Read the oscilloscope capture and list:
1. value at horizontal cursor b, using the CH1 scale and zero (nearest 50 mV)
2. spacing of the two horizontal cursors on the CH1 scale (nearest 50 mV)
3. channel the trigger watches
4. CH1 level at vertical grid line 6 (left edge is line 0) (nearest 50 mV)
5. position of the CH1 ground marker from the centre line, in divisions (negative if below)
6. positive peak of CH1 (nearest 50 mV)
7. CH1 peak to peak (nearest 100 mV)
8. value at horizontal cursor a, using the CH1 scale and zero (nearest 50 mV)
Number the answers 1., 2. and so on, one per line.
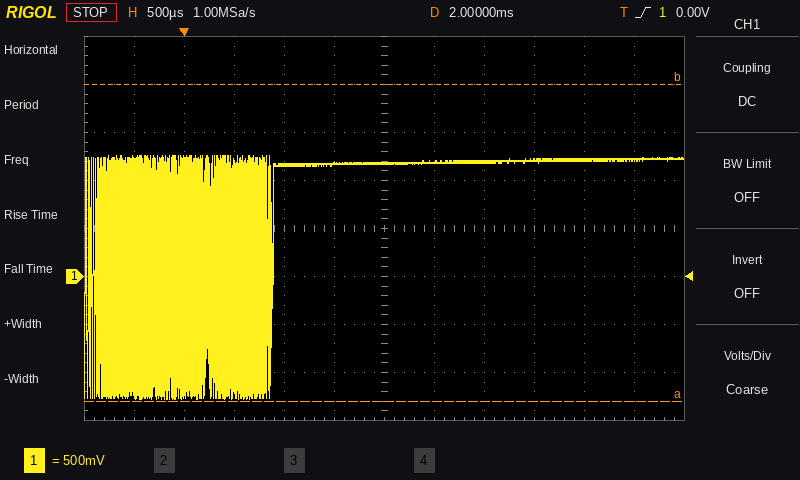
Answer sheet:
1. 2.00 V
2. 3.30 V
3. CH1
4. 1.20 V
5. -1.0 div
6. 1.25 V
7. 2.50 V
8. -1.30 V
